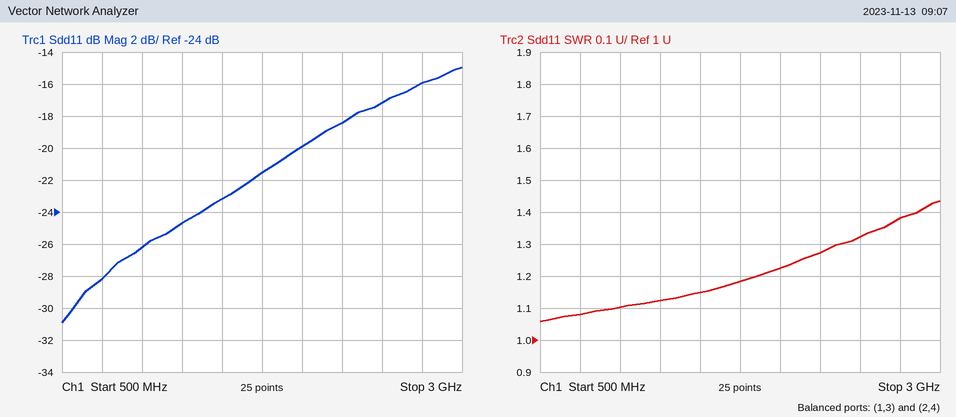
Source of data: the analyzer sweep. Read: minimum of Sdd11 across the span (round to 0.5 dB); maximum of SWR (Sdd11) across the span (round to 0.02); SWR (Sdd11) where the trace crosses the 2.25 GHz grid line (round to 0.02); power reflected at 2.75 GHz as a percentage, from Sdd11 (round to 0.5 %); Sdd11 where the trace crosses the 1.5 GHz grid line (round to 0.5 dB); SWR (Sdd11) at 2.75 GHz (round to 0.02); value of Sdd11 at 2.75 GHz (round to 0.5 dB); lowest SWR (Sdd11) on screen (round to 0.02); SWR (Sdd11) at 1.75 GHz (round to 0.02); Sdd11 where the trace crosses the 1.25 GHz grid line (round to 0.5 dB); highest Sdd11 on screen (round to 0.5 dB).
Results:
-31.0 dB
1.44
1.28
2.5 %
-23.0 dB
1.38
-16.0 dB
1.06
1.18
-24.5 dB
-15.0 dB
